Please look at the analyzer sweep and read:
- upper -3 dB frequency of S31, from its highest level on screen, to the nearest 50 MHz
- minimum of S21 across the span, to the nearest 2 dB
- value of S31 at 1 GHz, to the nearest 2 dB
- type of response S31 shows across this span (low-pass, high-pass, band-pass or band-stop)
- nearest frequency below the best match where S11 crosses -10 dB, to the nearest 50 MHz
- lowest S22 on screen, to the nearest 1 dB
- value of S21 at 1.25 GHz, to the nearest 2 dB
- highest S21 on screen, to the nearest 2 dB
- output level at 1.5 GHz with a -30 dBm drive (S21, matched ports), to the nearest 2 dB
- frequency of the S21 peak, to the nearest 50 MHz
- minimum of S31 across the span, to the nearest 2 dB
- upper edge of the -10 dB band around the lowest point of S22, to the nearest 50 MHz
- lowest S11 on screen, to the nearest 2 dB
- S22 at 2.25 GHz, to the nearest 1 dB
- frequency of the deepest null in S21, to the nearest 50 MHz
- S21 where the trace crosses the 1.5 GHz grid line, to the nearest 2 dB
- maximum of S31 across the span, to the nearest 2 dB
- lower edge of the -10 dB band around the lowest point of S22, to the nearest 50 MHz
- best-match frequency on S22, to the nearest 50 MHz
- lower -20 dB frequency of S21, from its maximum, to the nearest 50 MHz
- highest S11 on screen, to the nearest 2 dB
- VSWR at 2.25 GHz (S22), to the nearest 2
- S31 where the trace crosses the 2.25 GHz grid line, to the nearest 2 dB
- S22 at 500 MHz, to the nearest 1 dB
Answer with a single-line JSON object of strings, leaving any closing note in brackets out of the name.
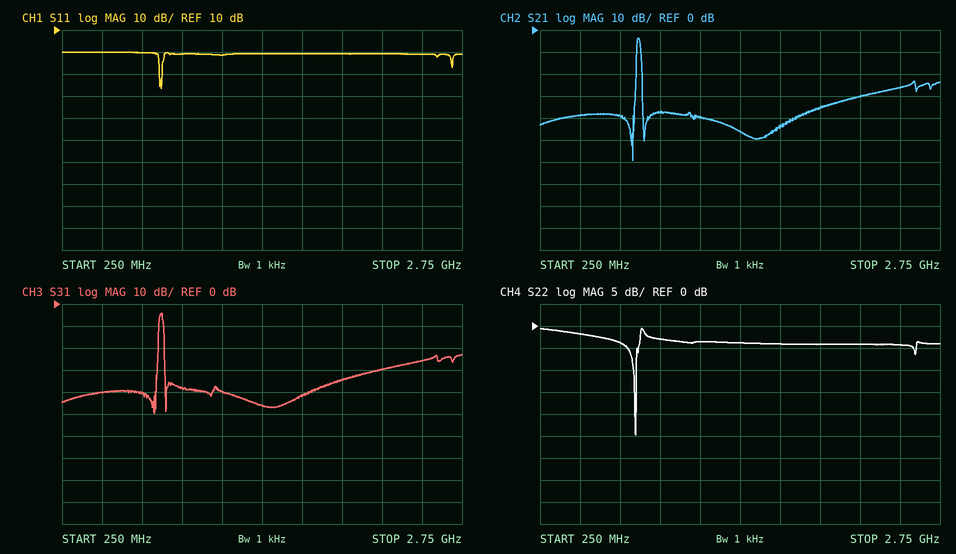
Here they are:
{"upper -3 dB frequency of S31, from its highest level on screen, to the nearest 50 MHz": "900 MHz", "minimum of S21 across the span, to the nearest 2 dB": "-60 dB", "value of S31 at 1 GHz, to the nearest 2 dB": "-38 dB", "type of response S31 shows across this span": "band-pass", "nearest frequency below the best match where S11 crosses -10 dB, to the nearest 50 MHz": "850 MHz", "lowest S22 on screen, to the nearest 1 dB": "-25 dB", "value of S21 at 1.25 GHz, to the nearest 2 dB": "-40 dB", "highest S21 on screen, to the nearest 2 dB": "-4 dB", "output level at 1.5 GHz with a -30 dBm drive (S21, matched ports), to the nearest 2 dB": "-76 dBm", "frequency of the S21 peak, to the nearest 50 MHz": "850 MHz", "minimum of S31 across the span, to the nearest 2 dB": "-50 dB", "upper edge of the -10 dB band around the lowest point of S22, to the nearest 50 MHz": "850 MHz", "lowest S11 on screen, to the nearest 2 dB": "-16 dB", "S22 at 2.25 GHz, to the nearest 1 dB": "-4 dB", "frequency of the deepest null in S21, to the nearest 50 MHz": "850 MHz", "S21 where the trace crosses the 1.5 GHz grid line, to the nearest 2 dB": "-46 dB", "maximum of S31 across the span, to the nearest 2 dB": "-4 dB", "lower edge of the -10 dB band around the lowest point of S22, to the nearest 50 MHz": "850 MHz", "best-match frequency on S22, to the nearest 50 MHz": "850 MHz", "lower -20 dB frequency of S21, from its maximum, to the nearest 50 MHz": "850 MHz", "highest S11 on screen, to the nearest 2 dB": "0 dB", "VSWR at 2.25 GHz (S22), to the nearest 2": "4", "S31 where the trace crosses the 2.25 GHz grid line, to the nearest 2 dB": "-30 dB", "S22 at 500 MHz, to the nearest 1 dB": "-2 dB"}
